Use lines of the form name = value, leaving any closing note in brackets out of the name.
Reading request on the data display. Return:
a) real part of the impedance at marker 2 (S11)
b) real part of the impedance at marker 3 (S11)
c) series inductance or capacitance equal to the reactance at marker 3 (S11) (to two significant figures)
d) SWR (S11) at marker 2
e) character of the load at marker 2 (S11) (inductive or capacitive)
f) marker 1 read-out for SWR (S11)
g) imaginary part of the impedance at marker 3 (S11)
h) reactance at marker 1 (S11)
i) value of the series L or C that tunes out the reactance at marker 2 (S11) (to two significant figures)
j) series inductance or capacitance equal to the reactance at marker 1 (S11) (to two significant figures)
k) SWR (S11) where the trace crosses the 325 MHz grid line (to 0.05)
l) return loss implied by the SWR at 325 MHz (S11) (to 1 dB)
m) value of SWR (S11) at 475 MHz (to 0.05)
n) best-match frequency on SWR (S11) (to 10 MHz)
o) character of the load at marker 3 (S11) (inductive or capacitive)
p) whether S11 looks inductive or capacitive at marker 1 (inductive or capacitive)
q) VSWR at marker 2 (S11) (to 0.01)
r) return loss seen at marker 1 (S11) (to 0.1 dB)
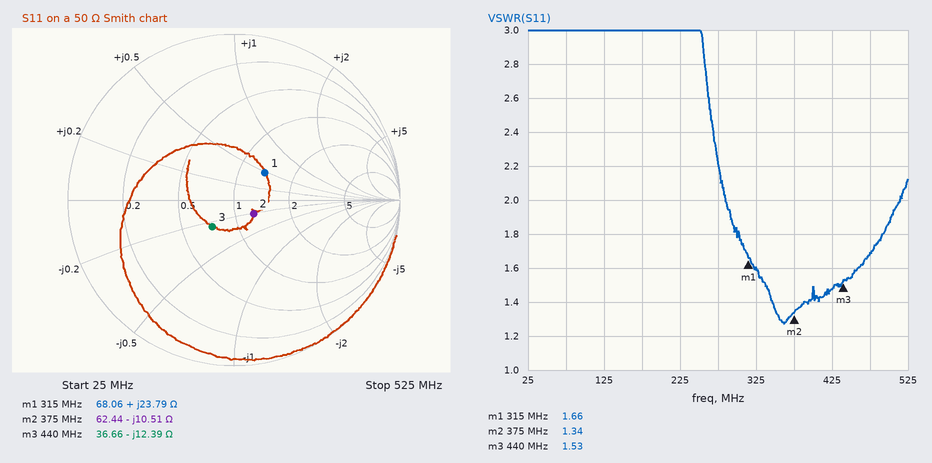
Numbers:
real part of the impedance at marker 2 = 62.44 Ω
real part of the impedance at marker 3 = 36.66 Ω
series inductance or capacitance equal to the reactance at marker 3 (S11) = 29 pF
SWR (S11) at marker 2 = 1.34
character of the load at marker 2 (S11) = capacitive
marker 1 read-out for SWR = 1.66
imaginary part of the impedance at marker 3 = -12.39 Ω
reactance at marker 1 = +23.79 Ω
value of the series L or C that tunes out the reactance at marker 2 (S11) = 4.5 nH
series inductance or capacitance equal to the reactance at marker 1 (S11) = 12 nH
SWR (S11) where the trace crosses the 325 MHz grid line = 1.60
return loss implied by the SWR at 325 MHz (S11) = 13 dB
value of SWR (S11) at 475 MHz = 1.70
best-match frequency on SWR (S11) = 360 MHz
character of the load at marker 3 (S11) = capacitive
whether S11 looks inductive or capacitive at marker 1 = inductive
VSWR at marker 2 (S11) = 1.34
return loss seen at marker 1 (S11) = 12.1 dB
